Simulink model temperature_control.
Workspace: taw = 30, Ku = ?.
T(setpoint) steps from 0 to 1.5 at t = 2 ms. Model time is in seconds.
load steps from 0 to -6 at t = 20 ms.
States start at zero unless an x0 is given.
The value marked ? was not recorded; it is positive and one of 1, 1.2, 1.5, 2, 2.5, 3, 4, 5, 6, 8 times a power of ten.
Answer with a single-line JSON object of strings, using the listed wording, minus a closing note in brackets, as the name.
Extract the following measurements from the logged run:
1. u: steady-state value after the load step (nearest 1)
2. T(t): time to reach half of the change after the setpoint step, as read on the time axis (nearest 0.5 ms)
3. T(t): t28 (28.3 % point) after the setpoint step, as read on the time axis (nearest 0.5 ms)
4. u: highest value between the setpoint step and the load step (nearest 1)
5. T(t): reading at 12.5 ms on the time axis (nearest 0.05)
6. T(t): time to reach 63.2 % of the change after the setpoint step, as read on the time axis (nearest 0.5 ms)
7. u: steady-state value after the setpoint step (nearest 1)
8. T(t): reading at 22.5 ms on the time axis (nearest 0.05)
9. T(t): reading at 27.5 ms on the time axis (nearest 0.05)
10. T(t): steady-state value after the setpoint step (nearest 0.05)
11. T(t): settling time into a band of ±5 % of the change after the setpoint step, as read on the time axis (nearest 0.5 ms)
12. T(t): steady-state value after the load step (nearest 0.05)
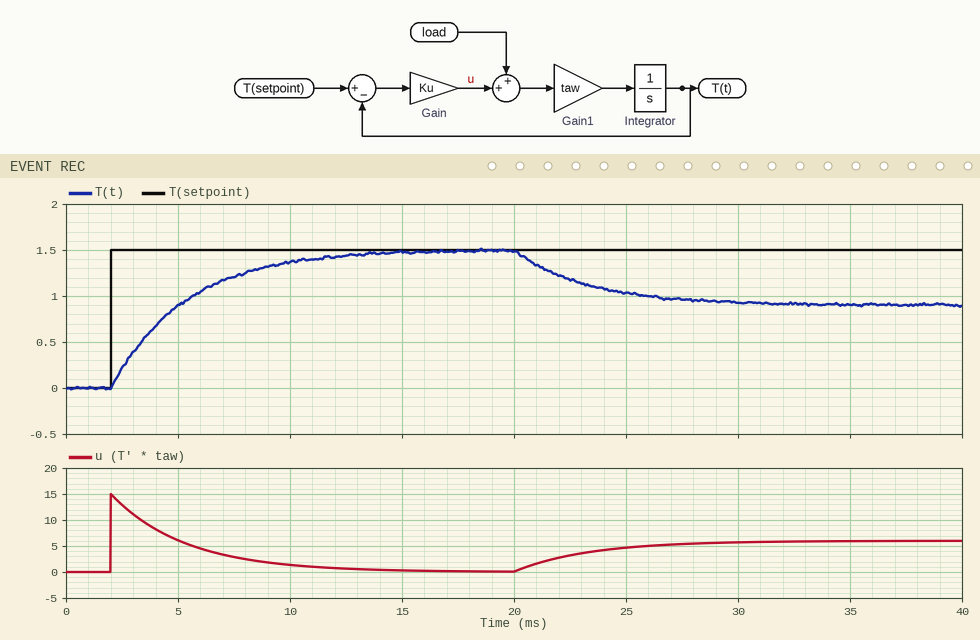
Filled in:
{"u: steady-state value after the load step": "6", "T(t): time to reach half of the change after the setpoint step, as read on the time axis": "4.5 ms", "T(t): t28 (28.3 % point) after the setpoint step, as read on the time axis": "3.0 ms", "u: highest value between the setpoint step and the load step": "15", "T(t): reading at 12.5 ms on the time axis": "1.45", "T(t): time to reach 63.2 % of the change after the setpoint step, as read on the time axis": "5.5 ms", "u: steady-state value after the setpoint step": "0", "T(t): reading at 22.5 ms on the time axis": "1.20", "T(t): reading at 27.5 ms on the time axis": "0.95", "T(t): steady-state value after the setpoint step": "1.50", "T(t): settling time into a band of ±5 % of the change after the setpoint step, as read on the time axis": "12.0 ms", "T(t): steady-state value after the load step": "0.90"}
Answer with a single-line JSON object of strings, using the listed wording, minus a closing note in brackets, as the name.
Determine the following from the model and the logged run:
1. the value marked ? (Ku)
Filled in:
{"the value marked ?": "10"}
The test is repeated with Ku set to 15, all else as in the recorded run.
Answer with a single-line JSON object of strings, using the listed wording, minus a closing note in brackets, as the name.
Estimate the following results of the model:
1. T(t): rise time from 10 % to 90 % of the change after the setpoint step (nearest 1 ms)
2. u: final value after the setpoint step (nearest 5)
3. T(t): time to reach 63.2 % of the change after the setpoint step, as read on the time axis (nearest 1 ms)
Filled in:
{"T(t): rise time from 10 % to 90 % of the change after the setpoint step": "5 ms", "u: final value after the setpoint step": "0", "T(t): time to reach 63.2 % of the change after the setpoint step, as read on the time axis": "4 ms"}
